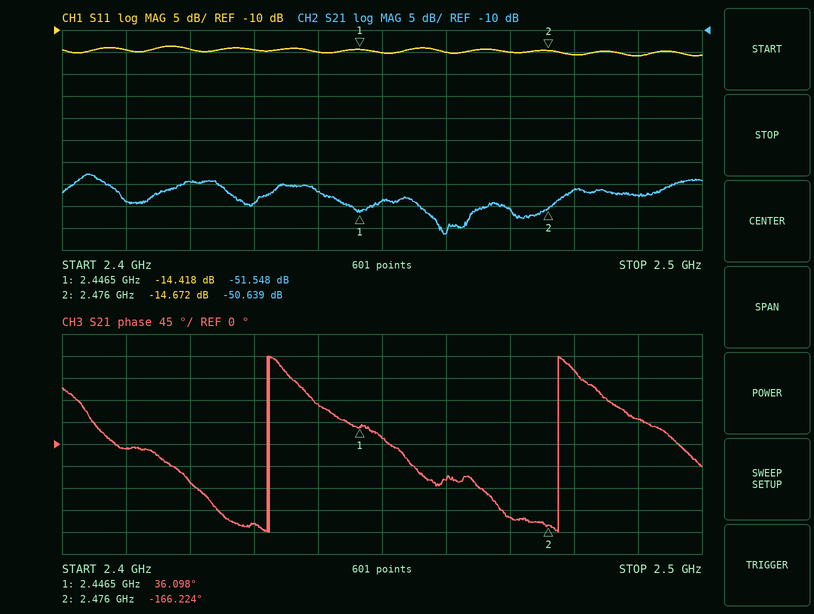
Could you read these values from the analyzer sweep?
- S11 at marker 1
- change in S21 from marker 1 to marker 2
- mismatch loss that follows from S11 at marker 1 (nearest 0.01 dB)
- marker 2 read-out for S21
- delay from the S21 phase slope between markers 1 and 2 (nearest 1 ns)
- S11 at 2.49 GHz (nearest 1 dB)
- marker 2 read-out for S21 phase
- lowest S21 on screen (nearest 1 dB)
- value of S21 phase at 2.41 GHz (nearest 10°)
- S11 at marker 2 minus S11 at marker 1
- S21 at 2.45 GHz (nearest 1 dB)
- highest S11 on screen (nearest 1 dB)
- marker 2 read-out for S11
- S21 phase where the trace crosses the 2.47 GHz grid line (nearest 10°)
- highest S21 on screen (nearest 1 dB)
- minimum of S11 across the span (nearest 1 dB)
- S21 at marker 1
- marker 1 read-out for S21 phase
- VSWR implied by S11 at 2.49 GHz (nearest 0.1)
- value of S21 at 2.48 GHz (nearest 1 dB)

-14.418 dB
0.909 dB
0.16 dB
-50.639 dB
19 ns
-16 dB
-166.224°
-56 dB
-10°
-0.254 dB
-49 dB
-14 dB
-14.672 dB
-150°
-43 dB
-16 dB
-51.548 dB
36.098°
1.4
-46 dB
